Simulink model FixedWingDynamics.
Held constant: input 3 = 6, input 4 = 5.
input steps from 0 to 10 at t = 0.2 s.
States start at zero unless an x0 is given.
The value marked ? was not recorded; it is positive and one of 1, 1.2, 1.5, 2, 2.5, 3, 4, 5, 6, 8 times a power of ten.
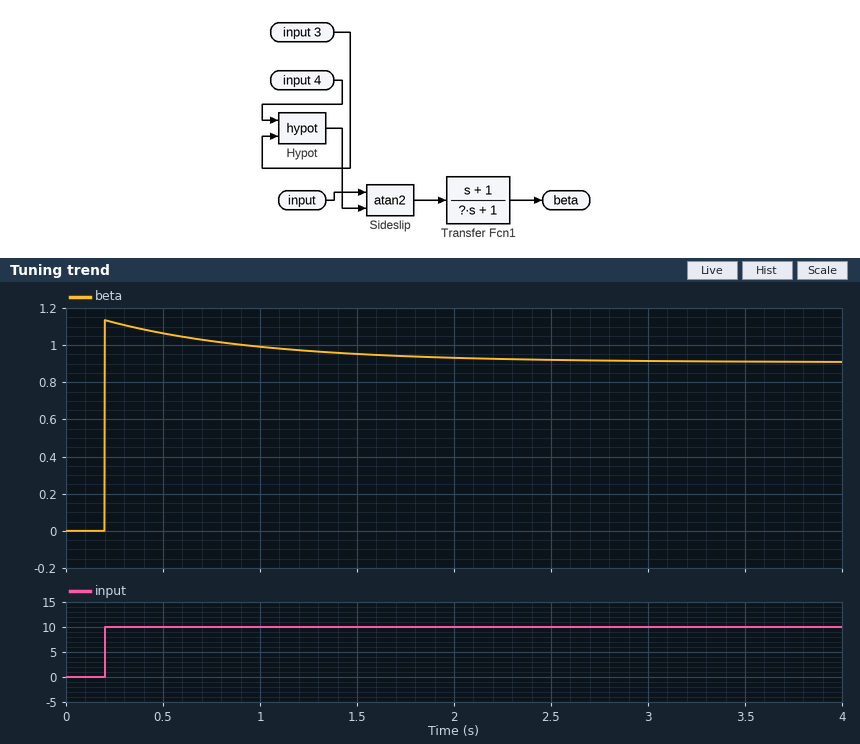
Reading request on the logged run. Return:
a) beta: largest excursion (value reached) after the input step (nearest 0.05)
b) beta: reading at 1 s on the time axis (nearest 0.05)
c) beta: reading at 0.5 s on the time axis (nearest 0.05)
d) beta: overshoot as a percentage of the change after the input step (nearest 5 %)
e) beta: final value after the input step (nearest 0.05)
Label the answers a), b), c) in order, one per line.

a) 1.15
b) 1.00
c) 1.05
d) 25 %
e) 0.90
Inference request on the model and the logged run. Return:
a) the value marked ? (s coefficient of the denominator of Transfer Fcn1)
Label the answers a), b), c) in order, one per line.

a) 0.8
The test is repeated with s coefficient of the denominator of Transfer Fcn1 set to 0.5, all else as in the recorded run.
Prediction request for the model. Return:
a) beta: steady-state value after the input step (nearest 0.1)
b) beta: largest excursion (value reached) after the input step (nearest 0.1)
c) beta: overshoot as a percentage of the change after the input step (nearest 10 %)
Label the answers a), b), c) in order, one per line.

a) 0.9
b) 1.8
c) 100 %
